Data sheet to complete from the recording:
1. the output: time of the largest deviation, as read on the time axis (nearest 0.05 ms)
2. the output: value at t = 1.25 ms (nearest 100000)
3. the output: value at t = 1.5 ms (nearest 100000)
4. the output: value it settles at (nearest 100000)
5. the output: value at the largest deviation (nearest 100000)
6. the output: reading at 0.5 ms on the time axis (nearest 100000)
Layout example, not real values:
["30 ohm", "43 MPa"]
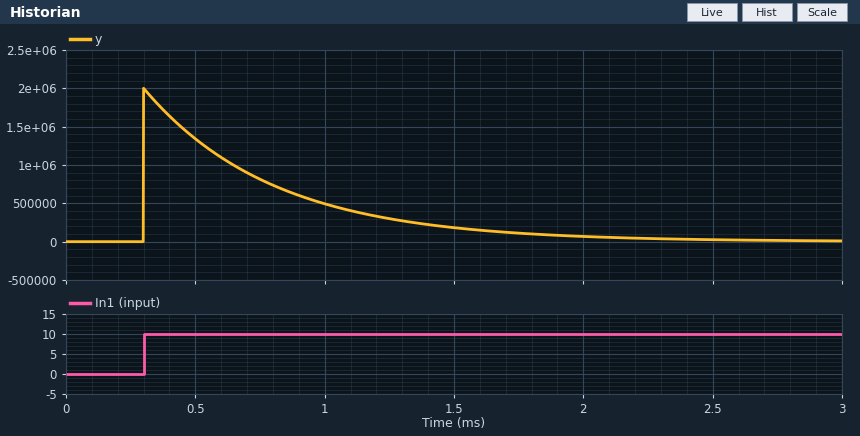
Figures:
["0.30 ms", "300000", "200000", "0", "2000000", "1300000"]
